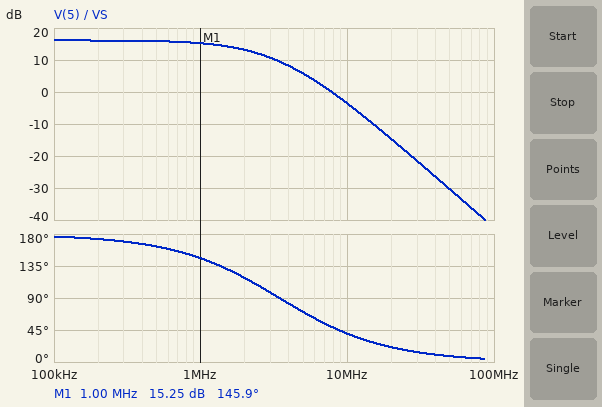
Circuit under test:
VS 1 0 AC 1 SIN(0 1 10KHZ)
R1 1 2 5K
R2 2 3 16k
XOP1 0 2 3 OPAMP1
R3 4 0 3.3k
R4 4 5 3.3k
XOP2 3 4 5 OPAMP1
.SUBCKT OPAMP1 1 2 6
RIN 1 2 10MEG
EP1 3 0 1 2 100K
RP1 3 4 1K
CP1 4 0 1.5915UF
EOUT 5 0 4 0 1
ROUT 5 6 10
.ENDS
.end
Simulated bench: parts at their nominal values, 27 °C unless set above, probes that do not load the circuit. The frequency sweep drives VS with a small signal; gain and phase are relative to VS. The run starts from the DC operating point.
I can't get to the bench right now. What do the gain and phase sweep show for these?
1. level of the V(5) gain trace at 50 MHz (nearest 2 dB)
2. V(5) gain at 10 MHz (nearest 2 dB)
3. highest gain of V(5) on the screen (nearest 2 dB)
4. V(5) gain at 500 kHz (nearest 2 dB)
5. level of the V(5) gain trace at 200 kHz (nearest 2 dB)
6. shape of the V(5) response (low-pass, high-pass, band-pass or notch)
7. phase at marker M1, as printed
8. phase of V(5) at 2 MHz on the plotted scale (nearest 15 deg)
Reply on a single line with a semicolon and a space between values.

-30 dB; -4 dB; 16 dB; 16 dB; 16 dB; low-pass; 145.9 deg; 120 deg
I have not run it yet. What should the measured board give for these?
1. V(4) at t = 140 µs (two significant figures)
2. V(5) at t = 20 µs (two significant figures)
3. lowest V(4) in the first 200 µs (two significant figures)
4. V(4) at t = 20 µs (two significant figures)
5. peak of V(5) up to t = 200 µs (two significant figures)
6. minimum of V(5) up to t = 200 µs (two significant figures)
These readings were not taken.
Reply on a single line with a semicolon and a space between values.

-1.9 V; -6.1 V; -3.2 V; -3.0 V; 6.4 V; -6.4 V
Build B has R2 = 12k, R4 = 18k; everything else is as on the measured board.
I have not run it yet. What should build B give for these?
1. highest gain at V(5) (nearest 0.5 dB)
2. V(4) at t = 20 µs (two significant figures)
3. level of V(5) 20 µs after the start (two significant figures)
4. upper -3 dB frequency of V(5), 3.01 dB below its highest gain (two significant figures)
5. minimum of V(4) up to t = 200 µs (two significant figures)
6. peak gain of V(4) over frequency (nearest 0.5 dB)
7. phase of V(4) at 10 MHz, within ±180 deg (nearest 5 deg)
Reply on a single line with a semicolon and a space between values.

24.0 dB; -2.3 V; -15 V; 1.3 MHz; -2.4 V; 7.5 dB; 25 deg
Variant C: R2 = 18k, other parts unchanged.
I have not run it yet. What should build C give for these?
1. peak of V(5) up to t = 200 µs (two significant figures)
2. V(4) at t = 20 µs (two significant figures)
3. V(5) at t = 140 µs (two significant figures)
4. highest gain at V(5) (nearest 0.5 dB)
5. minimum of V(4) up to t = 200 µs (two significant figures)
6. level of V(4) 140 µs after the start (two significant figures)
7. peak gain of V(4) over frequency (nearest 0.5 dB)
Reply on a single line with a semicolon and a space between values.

7.2 V; -3.4 V; -4.3 V; 17.0 dB; -3.6 V; -2.1 V; 11.0 dB
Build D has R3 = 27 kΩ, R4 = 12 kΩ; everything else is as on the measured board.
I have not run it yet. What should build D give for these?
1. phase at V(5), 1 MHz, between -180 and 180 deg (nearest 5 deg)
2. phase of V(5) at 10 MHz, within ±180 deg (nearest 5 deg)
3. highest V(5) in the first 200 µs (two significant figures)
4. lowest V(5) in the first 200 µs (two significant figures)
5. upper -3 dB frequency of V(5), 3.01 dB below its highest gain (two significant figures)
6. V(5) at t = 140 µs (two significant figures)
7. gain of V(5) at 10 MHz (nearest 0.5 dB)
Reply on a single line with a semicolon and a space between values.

150 deg; 50 deg; 4.6 V; -4.6 V; 2.2 MHz; -2.7 V; -4.5 dB
